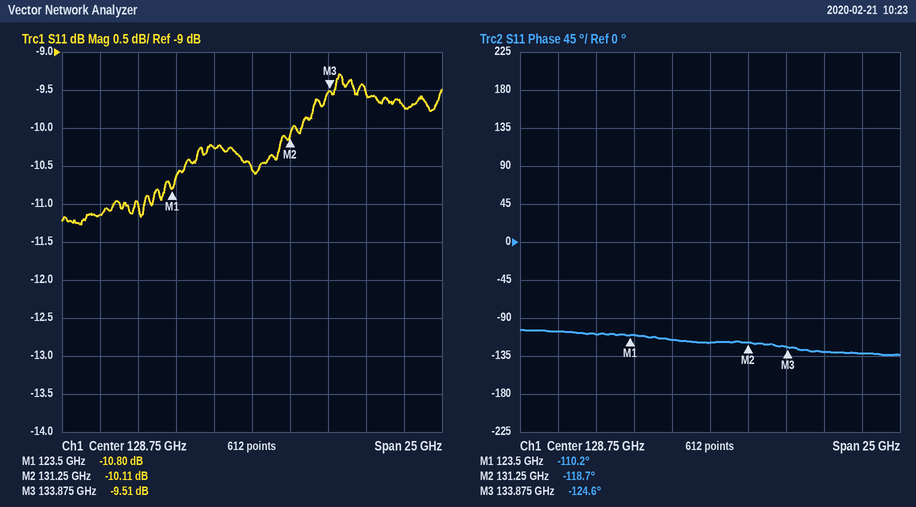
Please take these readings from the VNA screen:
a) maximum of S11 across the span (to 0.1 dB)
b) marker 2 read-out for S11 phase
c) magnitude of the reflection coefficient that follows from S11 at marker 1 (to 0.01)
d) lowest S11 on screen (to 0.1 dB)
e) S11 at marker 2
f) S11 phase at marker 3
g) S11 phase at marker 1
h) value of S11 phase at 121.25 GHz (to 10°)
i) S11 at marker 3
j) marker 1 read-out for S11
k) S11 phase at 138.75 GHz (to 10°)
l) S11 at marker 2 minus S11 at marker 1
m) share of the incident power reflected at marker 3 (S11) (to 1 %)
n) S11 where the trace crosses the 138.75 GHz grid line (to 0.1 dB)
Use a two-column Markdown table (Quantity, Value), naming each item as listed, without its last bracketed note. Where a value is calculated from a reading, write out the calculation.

| Quantity | Value |
|---|---|
| maximum of S11 across the span | -9.3 dB |
| marker 2 read-out for S11 phase | -118.7° |
| magnitude of the reflection coefficient that follows from S11 at marker 1 | 10^(-10.8/20) ≈ 0.29 |
| lowest S11 on screen | -11.3 dB |
| S11 at marker 2 | -10.11 dB |
| S11 phase at marker 3 | -124.6° |
| S11 phase at marker 1 | -110.2° |
| value of S11 phase at 121.25 GHz | -110° |
| S11 at marker 3 | -9.51 dB |
| marker 1 read-out for S11 | -10.80 dB |
| S11 phase at 138.75 GHz | -130° |
| S11 at marker 2 minus S11 at marker 1 | -10.11 − (-10.8) = 0.69 dB |
| share of the incident power reflected at marker 3 (S11) | 10^(-9.51/10) ≈ 11 % |
| S11 where the trace crosses the 138.75 GHz grid line | -9.7 dB |
